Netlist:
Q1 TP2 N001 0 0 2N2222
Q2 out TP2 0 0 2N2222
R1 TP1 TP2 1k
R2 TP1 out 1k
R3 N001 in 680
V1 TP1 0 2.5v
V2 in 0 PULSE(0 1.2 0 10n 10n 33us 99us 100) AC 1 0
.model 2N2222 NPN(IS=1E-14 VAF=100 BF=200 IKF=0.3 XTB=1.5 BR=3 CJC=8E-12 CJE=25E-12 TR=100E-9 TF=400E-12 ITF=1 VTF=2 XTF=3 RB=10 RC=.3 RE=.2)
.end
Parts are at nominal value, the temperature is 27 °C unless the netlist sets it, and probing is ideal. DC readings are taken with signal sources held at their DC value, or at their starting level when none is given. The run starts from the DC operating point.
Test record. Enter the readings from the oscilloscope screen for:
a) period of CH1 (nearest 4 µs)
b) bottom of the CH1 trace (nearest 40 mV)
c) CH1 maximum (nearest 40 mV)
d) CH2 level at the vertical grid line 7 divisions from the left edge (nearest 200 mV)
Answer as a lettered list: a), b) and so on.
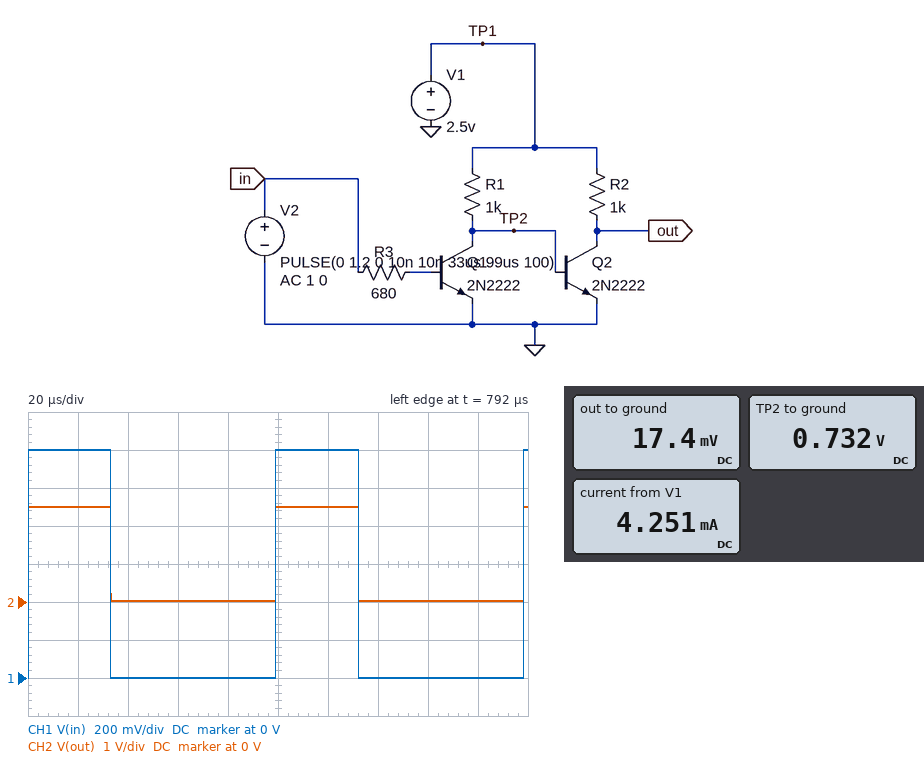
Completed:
a) 100 µs
b) 0 V
c) 1.20 V
d) 0 V
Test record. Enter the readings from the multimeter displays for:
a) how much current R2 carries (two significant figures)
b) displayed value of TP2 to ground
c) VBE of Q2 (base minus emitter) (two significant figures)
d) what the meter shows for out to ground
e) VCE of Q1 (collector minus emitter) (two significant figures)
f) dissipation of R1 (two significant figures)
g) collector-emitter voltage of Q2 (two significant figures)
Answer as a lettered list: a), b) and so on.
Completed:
a) 2.5 mA
b) 0.732 V
c) 730 mV
d) 17.4 mV
e) 730 mV
f) 3.1 mW
g) 17 mV
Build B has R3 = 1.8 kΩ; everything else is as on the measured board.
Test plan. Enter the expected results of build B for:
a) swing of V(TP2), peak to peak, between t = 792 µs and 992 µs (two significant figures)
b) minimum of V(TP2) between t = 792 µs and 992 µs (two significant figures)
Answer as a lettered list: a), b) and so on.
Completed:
a) 700 mV
b) 36 mV
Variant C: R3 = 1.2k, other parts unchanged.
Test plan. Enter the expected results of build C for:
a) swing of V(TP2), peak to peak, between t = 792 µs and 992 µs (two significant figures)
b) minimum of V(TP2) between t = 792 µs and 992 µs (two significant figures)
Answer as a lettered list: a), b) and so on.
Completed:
a) 710 mV
b) 27 mV
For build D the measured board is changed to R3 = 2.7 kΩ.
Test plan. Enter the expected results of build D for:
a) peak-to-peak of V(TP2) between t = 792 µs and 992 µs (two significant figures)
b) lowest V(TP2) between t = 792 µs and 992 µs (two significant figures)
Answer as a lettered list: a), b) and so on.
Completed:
a) 690 mV
b) 45 mV
